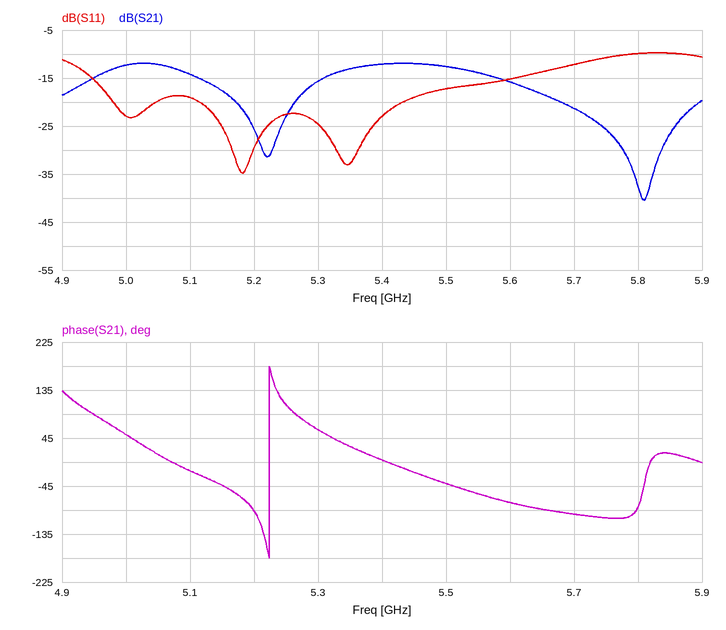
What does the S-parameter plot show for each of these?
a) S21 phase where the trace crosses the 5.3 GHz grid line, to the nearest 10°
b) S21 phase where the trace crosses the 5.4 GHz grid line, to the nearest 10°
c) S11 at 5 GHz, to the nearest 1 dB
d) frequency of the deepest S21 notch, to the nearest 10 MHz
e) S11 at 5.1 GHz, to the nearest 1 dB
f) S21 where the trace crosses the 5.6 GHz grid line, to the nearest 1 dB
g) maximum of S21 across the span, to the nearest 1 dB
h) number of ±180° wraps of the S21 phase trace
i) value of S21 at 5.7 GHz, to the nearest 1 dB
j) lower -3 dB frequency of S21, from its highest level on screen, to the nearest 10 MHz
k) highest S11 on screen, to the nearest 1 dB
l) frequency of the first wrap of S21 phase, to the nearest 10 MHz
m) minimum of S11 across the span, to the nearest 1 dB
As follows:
60°
0°
-23 dB
5.81 GHz
-19 dB
-16 dB
-12 dB
1
-21 dB
4.95 GHz
-10 dB
5.22 GHz
-35 dB
